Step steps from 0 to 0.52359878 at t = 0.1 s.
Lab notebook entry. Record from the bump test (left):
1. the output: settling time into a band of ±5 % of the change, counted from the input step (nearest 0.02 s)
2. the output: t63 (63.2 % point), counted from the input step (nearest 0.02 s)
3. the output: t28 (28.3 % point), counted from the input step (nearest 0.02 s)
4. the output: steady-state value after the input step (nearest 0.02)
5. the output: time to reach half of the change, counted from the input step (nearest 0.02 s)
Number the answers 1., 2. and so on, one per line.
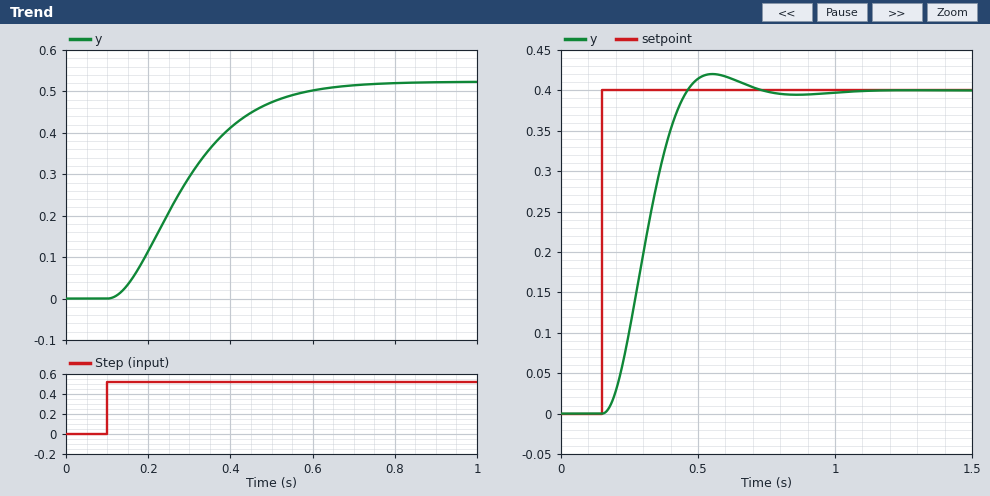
1. 0.48 s
2. 0.22 s
3. 0.12 s
4. 0.52
5. 0.18 s
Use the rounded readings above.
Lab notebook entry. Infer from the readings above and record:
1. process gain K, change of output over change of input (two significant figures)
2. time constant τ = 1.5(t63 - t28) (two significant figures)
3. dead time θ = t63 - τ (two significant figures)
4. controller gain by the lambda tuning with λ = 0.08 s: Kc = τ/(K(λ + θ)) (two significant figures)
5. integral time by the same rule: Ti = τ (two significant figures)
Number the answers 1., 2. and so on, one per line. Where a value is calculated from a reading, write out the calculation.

1. (0.52 - 0) / 0.523599 = 0.99
2. 1.5 × (0.22 - 0.12) = 0.15 s
3. 0.22 - 0.15 = 0.070 s
4. 0.15 / (0.99 × (0.08 + 0.07)) = 1.0
5. 0.15 s
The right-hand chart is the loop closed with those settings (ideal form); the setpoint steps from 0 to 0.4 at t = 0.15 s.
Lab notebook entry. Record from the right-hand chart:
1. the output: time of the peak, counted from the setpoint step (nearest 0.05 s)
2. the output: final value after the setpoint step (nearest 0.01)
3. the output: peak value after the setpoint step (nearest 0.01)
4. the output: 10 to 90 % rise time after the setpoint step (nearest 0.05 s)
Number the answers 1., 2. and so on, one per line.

1. 0.40 s
2. 0.40
3. 0.42
4. 0.20 s
